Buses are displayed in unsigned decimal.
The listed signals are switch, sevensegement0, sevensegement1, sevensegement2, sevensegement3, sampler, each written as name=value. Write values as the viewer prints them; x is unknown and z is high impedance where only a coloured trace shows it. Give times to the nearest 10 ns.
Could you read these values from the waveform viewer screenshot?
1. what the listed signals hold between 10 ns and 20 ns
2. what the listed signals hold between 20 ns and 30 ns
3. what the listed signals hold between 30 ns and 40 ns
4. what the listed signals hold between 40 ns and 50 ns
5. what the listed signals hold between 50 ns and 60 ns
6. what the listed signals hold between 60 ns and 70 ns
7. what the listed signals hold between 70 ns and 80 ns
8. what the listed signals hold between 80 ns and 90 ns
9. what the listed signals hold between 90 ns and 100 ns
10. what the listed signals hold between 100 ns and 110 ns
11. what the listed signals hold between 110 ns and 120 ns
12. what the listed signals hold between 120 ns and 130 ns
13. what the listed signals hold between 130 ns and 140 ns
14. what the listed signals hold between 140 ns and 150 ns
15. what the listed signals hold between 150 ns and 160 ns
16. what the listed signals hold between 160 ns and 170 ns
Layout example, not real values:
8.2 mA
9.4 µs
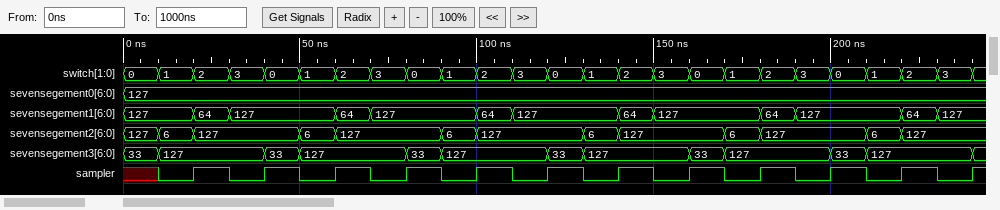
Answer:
switch=1, sevensegement0=127, sevensegement1=127, sevensegement2=6, sevensegement3=127, sampler=0
switch=2, sevensegement0=127, sevensegement1=64, sevensegement2=127, sevensegement3=127, sampler=1
switch=3, sevensegement0=127, sevensegement1=127, sevensegement2=127, sevensegement3=127, sampler=0
switch=0, sevensegement0=127, sevensegement1=127, sevensegement2=127, sevensegement3=33, sampler=1
switch=1, sevensegement0=127, sevensegement1=127, sevensegement2=6, sevensegement3=127, sampler=0
switch=2, sevensegement0=127, sevensegement1=64, sevensegement2=127, sevensegement3=127, sampler=1
switch=3, sevensegement0=127, sevensegement1=127, sevensegement2=127, sevensegement3=127, sampler=0
switch=0, sevensegement0=127, sevensegement1=127, sevensegement2=127, sevensegement3=33, sampler=1
switch=1, sevensegement0=127, sevensegement1=127, sevensegement2=6, sevensegement3=127, sampler=0
switch=2, sevensegement0=127, sevensegement1=64, sevensegement2=127, sevensegement3=127, sampler=1
switch=3, sevensegement0=127, sevensegement1=127, sevensegement2=127, sevensegement3=127, sampler=0
switch=0, sevensegement0=127, sevensegement1=127, sevensegement2=127, sevensegement3=33, sampler=1
switch=1, sevensegement0=127, sevensegement1=127, sevensegement2=6, sevensegement3=127, sampler=0
switch=2, sevensegement0=127, sevensegement1=64, sevensegement2=127, sevensegement3=127, sampler=1
switch=3, sevensegement0=127, sevensegement1=127, sevensegement2=127, sevensegement3=127, sampler=0
switch=0, sevensegement0=127, sevensegement1=127, sevensegement2=127, sevensegement3=33, sampler=1
